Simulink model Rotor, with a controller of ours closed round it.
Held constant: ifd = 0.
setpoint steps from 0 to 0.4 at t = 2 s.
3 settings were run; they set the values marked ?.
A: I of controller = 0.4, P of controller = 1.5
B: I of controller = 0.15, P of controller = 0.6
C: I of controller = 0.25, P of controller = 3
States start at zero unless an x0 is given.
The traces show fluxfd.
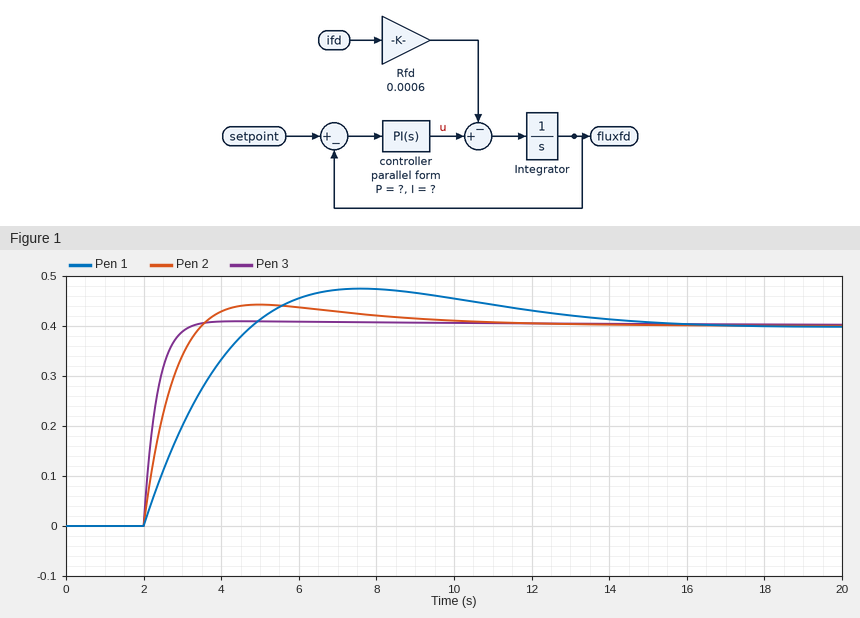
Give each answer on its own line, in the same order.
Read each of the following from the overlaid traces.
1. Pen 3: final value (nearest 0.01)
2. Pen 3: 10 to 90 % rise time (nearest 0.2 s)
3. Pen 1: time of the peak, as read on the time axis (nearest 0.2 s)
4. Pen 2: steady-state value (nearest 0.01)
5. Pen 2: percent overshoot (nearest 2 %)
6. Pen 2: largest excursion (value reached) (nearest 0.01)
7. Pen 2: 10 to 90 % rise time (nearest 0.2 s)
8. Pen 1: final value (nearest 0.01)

0.40
0.6 s
7.6 s
0.40
10 %
0.44
1.0 s
0.40
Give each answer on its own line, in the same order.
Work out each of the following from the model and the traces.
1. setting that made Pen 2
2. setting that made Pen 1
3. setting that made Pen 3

A
B
C
